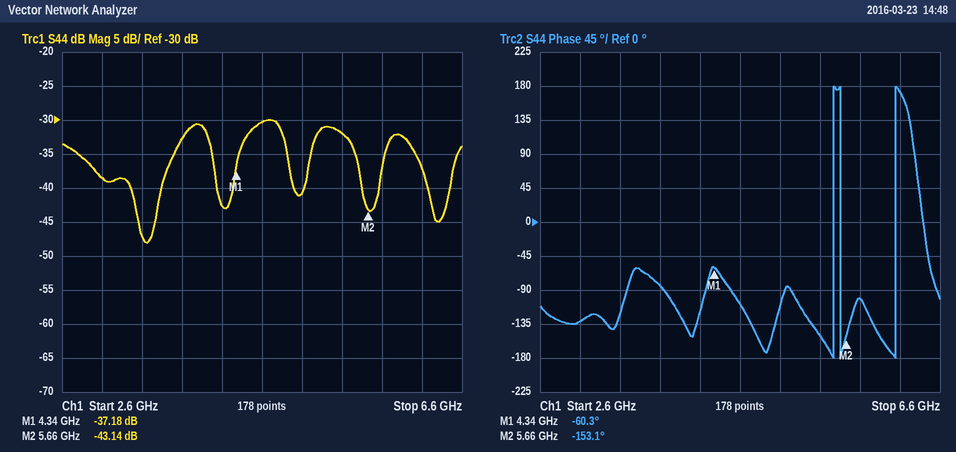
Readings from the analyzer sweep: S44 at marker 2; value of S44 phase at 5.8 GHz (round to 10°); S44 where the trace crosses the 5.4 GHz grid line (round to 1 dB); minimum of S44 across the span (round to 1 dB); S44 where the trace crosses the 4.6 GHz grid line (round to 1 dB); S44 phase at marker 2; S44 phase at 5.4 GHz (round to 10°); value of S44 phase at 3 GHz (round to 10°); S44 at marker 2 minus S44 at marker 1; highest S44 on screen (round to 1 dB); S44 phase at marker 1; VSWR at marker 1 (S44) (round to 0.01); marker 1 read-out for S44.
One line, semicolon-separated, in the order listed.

-43.14 dB; -100°; -32 dB; -48 dB; -30 dB; -153.1°; -150°; -130°; -5.96 dB; -30 dB; -60.3°; 1.03; -37.18 dB
